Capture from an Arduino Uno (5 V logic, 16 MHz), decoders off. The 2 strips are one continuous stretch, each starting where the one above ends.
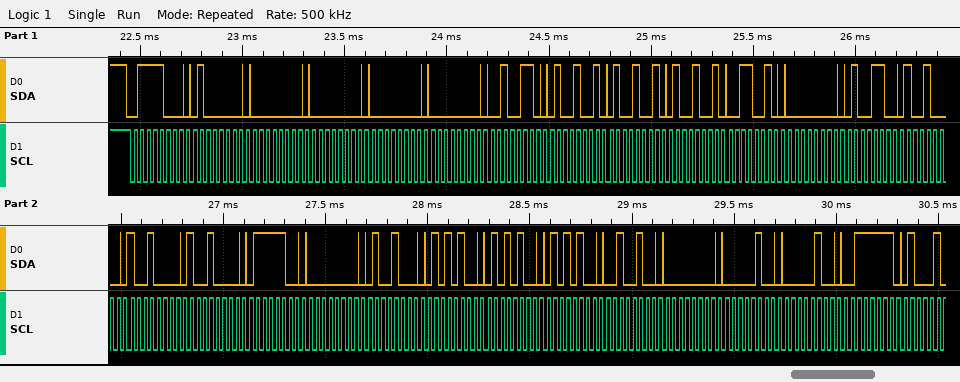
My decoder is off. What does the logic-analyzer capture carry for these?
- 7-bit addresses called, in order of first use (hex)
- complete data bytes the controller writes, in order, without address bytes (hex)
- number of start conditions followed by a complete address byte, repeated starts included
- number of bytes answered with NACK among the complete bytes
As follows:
0x3C
40 00 00 00 00 26 49 49 49 32 00 4C 90 90 90 7C 00 48 54 54 54 24 00 04 04 3F
1
0
